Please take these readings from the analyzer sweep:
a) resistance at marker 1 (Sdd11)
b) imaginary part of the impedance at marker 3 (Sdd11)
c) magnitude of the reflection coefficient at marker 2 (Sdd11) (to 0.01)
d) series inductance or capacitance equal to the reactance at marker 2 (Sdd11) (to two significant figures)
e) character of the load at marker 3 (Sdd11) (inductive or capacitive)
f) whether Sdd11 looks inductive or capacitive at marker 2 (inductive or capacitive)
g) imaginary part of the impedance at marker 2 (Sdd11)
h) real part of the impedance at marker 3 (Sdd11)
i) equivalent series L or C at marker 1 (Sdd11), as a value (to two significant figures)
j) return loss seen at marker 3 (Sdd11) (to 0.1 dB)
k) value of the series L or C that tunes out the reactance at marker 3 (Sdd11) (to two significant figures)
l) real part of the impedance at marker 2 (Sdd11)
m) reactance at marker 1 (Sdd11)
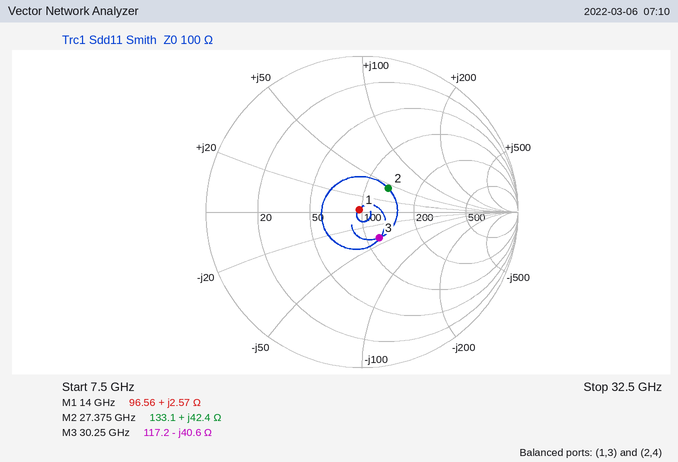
96.56 Ω
-40.6 Ω
0.23
250 pH
capacitive
inductive
+42.4 Ω
117.2 Ω
29 pH
14.0 dB
210 pH
133.1 Ω
+2.57 Ω
